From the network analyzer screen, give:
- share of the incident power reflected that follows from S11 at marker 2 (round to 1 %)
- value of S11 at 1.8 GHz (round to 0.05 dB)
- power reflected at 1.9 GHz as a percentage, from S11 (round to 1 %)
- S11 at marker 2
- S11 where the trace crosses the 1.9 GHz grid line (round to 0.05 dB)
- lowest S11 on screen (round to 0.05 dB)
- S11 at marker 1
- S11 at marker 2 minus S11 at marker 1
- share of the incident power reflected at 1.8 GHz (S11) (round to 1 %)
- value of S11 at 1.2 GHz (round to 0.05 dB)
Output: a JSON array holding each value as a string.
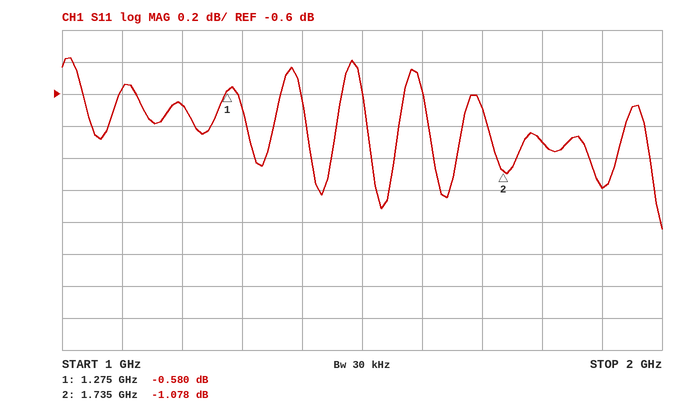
["78 %", "-0.90 dB", "76 %", "-1.078 dB", "-1.20 dB", "-1.45 dB", "-0.580 dB", "-0.498 dB", "81 %", "-0.65 dB"]
